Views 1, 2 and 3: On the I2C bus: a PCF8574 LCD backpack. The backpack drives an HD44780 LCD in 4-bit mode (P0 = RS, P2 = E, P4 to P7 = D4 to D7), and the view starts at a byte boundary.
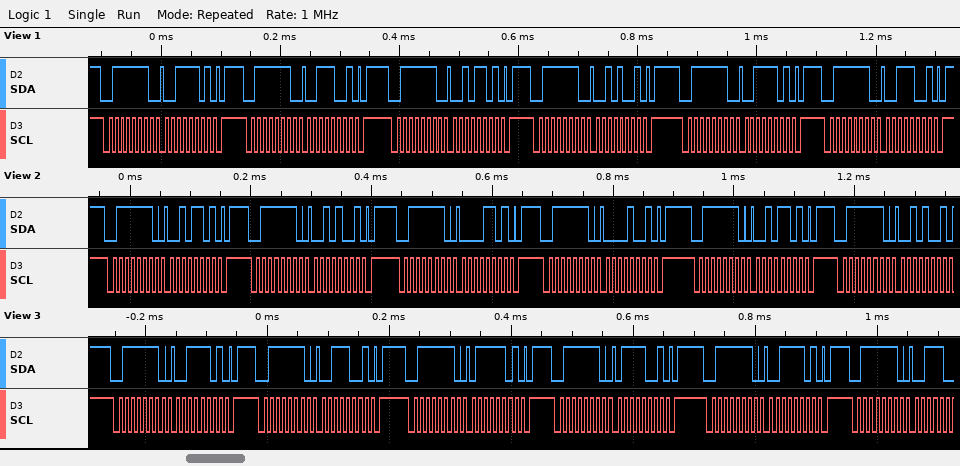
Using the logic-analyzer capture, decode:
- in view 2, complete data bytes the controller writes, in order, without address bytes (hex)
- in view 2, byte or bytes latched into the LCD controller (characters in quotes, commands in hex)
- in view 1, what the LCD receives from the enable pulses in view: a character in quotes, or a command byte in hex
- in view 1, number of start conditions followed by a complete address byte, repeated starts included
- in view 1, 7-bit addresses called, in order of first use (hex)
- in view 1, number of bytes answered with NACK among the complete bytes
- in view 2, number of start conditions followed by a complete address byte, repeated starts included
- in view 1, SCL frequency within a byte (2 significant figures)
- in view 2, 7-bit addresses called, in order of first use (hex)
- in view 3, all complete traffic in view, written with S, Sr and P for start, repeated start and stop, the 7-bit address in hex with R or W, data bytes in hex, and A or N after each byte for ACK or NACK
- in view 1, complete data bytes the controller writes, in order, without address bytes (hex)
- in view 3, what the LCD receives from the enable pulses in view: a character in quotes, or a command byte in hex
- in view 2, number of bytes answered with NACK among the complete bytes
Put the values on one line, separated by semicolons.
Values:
2D 29 0D 09 2D 29; ' '; '2'; 6; 0x3F; 0; 6; 100 kHz; 0x3F; S 3FW A 3D A P S 3FW A 39 A P S 3FW A 7D A P S 3FW A 79 A P S 3FW A 3D A P S 3FW A; 3D 39 2D 29 3D 39; '7'; 0
